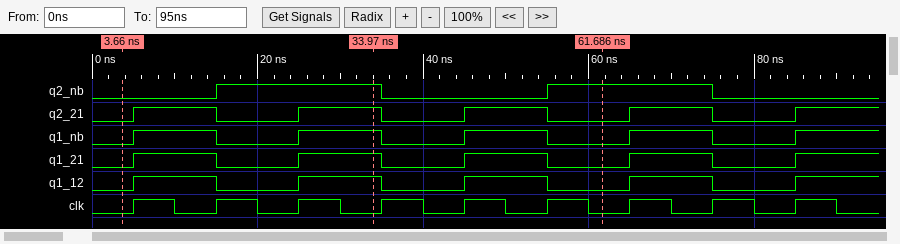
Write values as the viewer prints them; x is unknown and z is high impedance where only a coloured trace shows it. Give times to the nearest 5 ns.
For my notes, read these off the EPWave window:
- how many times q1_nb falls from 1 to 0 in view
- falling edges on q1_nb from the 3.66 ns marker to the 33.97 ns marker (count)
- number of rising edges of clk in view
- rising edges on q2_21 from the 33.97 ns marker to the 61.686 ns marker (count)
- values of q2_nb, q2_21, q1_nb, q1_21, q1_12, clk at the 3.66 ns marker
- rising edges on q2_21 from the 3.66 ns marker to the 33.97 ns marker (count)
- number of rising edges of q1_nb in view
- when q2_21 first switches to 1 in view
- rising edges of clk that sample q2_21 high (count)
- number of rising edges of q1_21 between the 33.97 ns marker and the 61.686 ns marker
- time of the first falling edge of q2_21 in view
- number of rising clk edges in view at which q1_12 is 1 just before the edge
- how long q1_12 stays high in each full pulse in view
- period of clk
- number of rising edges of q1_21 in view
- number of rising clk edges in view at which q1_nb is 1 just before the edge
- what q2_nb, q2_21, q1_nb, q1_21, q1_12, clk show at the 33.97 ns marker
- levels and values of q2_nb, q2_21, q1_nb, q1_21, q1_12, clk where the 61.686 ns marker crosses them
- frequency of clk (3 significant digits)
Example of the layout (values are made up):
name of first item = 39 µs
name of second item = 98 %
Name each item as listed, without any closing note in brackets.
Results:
how many times q1_nb falls from 1 to 0 in view = 4
falling edges on q1_nb from the 3.66 ns marker to the 33.97 ns marker = 1
number of rising edges of clk in view = 9
rising edges on q2_21 from the 33.97 ns marker to the 61.686 ns marker = 1
values of q2_nb, q2_21, q1_nb, q1_21, q1_12, clk at the 3.66 ns marker = q2_nb=0, q2_21=0, q1_nb=0, q1_21=0, q1_12=0, clk=0
rising edges on q2_21 from the 3.66 ns marker to the 33.97 ns marker = 2
number of rising edges of q1_nb in view = 5
when q2_21 first switches to 1 in view = 5 ns
rising edges of clk that sample q2_21 high = 4
number of rising edges of q1_21 between the 33.97 ns marker and the 61.686 ns marker = 1
time of the first falling edge of q2_21 in view = 15 ns
number of rising clk edges in view at which q1_12 is 1 just before the edge = 4
how long q1_12 stays high in each full pulse in view = 10 ns, 10 ns, 10 ns, 10 ns
period of clk = 10 ns
number of rising edges of q1_21 in view = 5
number of rising clk edges in view at which q1_nb is 1 just before the edge = 4
what q2_nb, q2_21, q1_nb, q1_21, q1_12, clk show at the 33.97 ns marker = q2_nb=1, q2_21=1, q1_nb=1, q1_21=1, q1_12=1, clk=0
levels and values of q2_nb, q2_21, q1_nb, q1_21, q1_12, clk where the 61.686 ns marker crosses them = q2_nb=1, q2_21=0, q1_nb=0, q1_21=0, q1_12=0, clk=0
frequency of clk = 100 MHz
